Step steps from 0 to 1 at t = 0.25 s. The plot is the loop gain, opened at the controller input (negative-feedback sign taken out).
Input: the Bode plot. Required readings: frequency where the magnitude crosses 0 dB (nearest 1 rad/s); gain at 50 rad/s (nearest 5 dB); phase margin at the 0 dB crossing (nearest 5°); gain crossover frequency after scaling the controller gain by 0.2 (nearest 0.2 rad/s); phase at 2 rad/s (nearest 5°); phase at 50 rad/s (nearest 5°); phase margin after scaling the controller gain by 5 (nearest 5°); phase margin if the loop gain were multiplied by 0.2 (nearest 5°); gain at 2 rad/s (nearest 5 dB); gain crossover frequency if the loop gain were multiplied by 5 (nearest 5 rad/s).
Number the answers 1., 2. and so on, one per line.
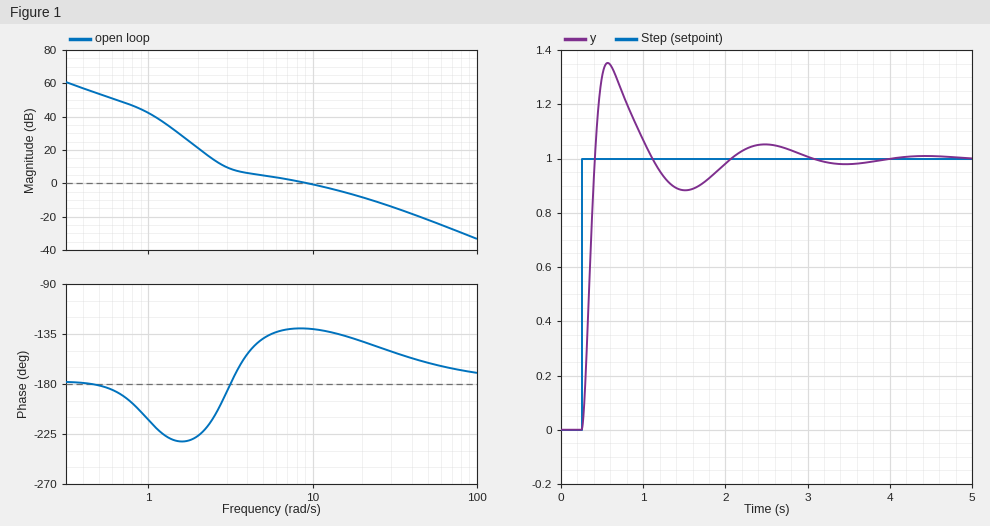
1. 9 rad/s
2. -20 dB
3. 50°
4. 2.6 rad/s
5. -225°
6. -160°
7. 30°
8. -30°
9. 20 dB
10. 30 rad/s
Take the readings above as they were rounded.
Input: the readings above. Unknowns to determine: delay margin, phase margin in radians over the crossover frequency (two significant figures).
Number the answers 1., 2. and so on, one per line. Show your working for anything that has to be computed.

1. 50 × π / 180 / 9 = 0.097 s
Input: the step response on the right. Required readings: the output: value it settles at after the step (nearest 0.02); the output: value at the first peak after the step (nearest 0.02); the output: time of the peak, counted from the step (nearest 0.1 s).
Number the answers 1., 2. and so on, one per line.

1. 1.00
2. 1.36
3. 0.3 s
